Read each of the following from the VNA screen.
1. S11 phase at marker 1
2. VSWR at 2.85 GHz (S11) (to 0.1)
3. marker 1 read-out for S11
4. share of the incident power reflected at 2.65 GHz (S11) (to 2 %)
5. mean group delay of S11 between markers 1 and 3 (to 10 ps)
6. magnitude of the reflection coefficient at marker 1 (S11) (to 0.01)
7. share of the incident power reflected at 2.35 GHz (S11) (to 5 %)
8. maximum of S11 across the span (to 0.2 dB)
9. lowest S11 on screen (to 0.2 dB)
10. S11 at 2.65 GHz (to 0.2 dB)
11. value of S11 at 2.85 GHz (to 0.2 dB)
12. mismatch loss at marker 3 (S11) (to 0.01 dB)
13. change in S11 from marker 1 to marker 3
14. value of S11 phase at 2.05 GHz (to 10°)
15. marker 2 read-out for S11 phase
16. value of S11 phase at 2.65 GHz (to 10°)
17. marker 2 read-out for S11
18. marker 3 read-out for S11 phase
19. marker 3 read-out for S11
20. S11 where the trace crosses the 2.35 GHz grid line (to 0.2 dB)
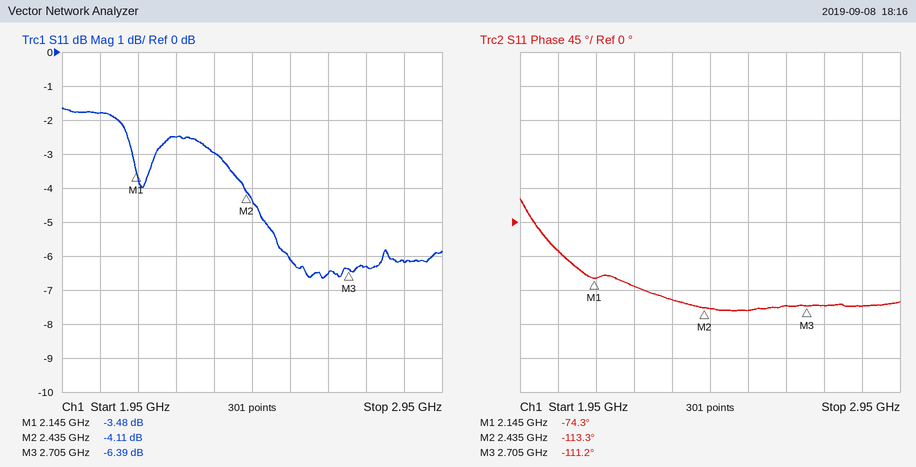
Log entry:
-74.3°
2.9
-3.48 dB
22 %
180 ps
0.67
50 %
-1.6 dB
-6.6 dB
-6.6 dB
-6.2 dB
1.13 dB
-2.91 dB
-40°
-113.3°
-110°
-4.11 dB
-111.2°
-6.39 dB
-3.0 dB
